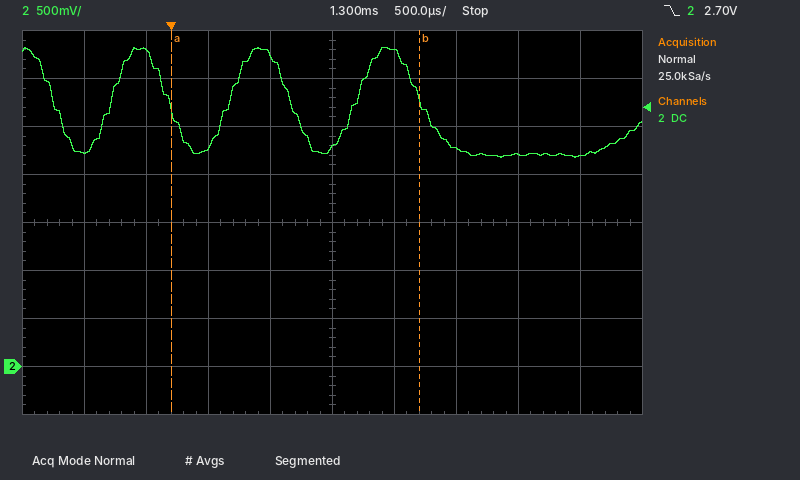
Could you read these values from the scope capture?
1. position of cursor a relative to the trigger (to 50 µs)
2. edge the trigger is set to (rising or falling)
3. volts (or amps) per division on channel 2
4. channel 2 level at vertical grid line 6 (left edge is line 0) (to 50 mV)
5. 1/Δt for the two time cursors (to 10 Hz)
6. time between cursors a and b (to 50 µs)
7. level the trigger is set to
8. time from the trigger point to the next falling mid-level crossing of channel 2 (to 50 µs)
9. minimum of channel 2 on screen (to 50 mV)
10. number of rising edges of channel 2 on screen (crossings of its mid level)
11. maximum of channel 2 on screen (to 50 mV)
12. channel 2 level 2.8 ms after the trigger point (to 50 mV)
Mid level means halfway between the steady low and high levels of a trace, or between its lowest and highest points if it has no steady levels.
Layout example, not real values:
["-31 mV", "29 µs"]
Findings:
["0 µs", "falling", "500 mV", "3.30 V", "500 Hz", "2.00 ms", "2.70 V", "950 µs", "2.20 V", "3", "3.30 V", "2.20 V"]
